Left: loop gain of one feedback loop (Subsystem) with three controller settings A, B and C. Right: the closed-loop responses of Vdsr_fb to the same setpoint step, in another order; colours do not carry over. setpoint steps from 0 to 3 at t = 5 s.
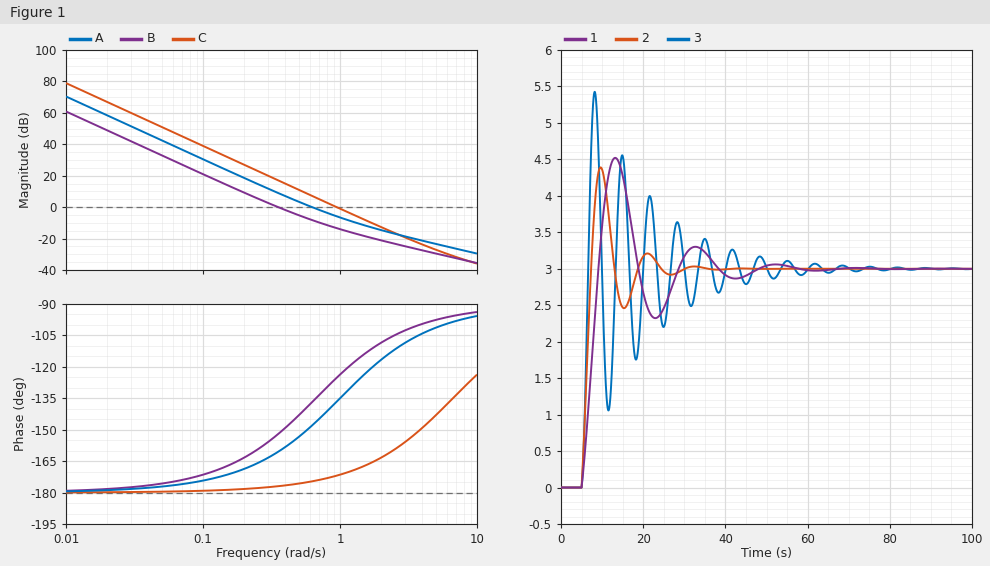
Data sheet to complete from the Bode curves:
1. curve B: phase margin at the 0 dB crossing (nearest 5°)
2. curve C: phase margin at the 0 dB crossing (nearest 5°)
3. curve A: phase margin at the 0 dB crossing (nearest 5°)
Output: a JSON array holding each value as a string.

["30°", "10°", "30°"]
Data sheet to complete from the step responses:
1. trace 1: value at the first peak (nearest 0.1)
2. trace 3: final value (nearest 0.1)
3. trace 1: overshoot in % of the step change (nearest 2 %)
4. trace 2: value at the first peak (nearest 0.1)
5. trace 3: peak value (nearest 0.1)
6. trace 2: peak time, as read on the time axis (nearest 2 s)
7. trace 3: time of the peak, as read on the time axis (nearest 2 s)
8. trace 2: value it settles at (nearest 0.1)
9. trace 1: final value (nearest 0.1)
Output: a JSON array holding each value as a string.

["4.5", "3.0", "50 %", "4.4", "5.4", "10 s", "8 s", "3.0", "3.0"]
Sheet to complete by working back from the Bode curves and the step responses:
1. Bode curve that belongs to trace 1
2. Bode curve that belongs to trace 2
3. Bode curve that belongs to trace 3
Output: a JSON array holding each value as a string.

["B", "A", "C"]
